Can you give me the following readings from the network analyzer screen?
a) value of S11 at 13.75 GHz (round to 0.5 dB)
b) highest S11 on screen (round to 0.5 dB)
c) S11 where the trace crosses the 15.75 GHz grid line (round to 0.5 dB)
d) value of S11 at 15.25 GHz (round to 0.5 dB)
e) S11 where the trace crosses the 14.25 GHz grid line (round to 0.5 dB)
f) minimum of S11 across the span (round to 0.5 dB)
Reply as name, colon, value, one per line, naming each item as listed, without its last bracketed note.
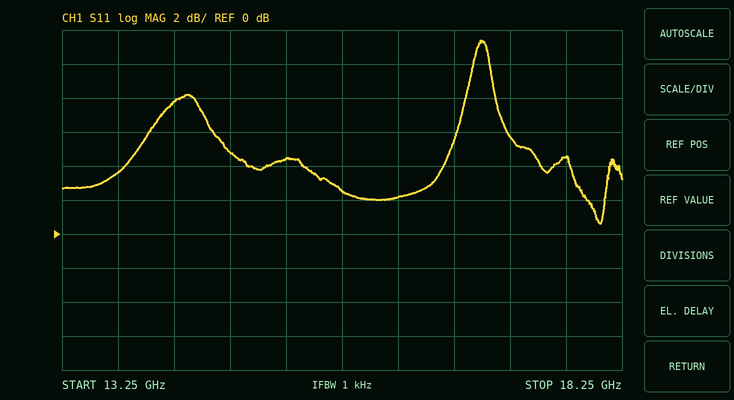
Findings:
value of S11 at 13.75 GHz: 3.5 dB
highest S11 on screen: 11.5 dB
S11 where the trace crosses the 15.75 GHz grid line: 2.5 dB
value of S11 at 15.25 GHz: 4.5 dB
S11 where the trace crosses the 14.25 GHz grid line: 8.0 dB
minimum of S11 across the span: 0.5 dB
